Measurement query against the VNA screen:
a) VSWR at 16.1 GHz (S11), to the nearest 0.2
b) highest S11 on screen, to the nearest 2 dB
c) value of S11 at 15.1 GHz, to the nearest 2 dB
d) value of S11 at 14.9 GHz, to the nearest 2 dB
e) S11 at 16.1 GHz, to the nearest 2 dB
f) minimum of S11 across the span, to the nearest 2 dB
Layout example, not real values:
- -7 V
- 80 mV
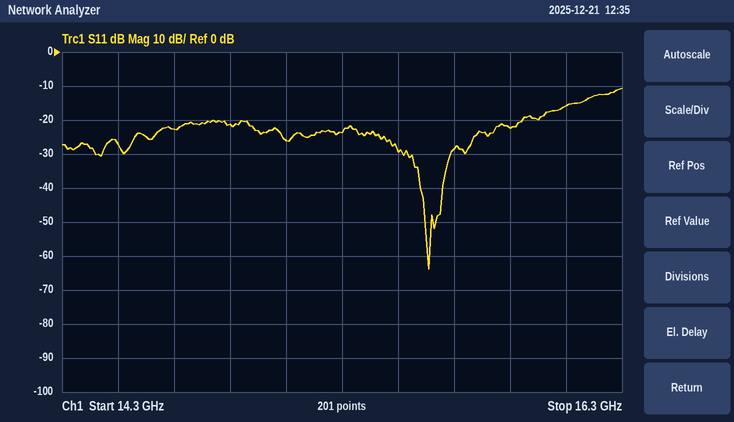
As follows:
- 1.4
- -10 dB
- -26 dB
- -22 dB
- -16 dB
- -64 dB
